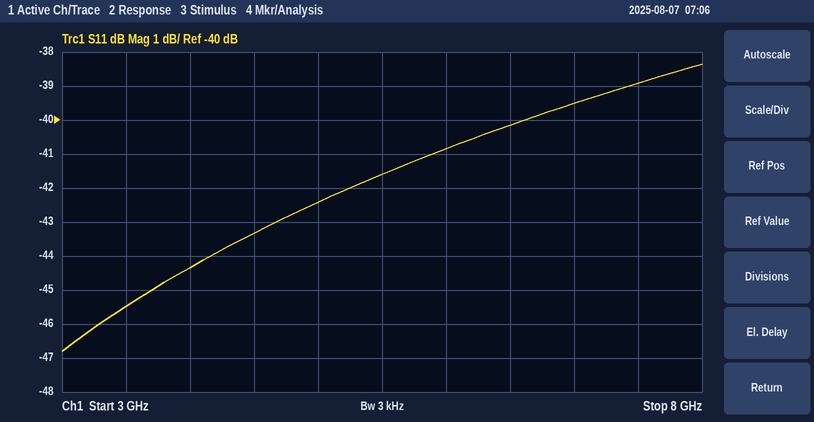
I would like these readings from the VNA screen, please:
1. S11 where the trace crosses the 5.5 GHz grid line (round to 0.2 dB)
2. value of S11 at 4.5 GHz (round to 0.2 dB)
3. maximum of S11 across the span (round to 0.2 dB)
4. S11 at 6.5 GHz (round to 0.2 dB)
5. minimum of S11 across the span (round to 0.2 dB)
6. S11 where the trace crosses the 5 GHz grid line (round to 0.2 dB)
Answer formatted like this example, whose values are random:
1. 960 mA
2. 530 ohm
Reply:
1. -41.6 dB
2. -43.4 dB
3. -38.4 dB
4. -40.2 dB
5. -46.8 dB
6. -42.4 dB
